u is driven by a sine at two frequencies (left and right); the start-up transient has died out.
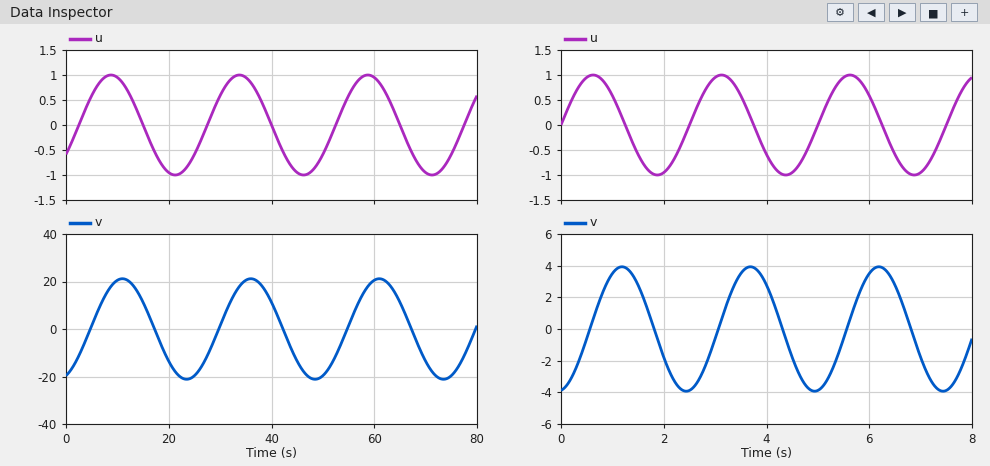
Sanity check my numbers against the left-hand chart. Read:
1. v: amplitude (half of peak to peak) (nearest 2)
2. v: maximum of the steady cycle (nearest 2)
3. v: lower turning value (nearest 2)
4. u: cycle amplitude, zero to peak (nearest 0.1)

22
22
-22
1.0
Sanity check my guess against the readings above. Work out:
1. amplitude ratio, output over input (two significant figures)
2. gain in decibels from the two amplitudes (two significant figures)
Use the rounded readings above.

22
27 dB
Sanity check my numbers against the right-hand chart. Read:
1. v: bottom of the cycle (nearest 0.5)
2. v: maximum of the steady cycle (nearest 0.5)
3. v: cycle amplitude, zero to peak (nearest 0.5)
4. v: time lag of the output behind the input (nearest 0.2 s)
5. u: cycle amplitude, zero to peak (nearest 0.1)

-4.0
4.0
4.0
0.6 s
1.0
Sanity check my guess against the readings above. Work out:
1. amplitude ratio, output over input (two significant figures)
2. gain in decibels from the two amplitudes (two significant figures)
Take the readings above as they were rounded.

4.0
12 dB
